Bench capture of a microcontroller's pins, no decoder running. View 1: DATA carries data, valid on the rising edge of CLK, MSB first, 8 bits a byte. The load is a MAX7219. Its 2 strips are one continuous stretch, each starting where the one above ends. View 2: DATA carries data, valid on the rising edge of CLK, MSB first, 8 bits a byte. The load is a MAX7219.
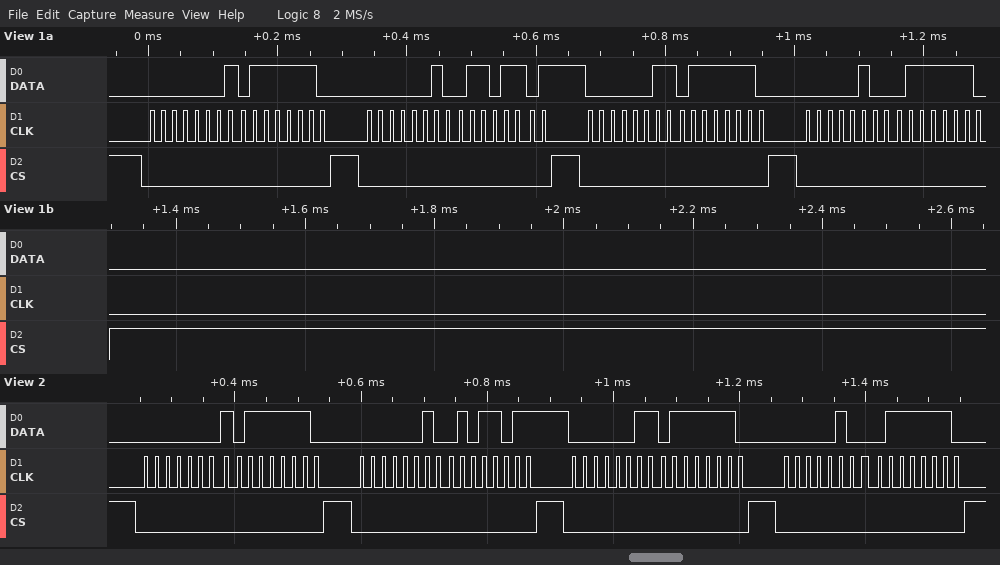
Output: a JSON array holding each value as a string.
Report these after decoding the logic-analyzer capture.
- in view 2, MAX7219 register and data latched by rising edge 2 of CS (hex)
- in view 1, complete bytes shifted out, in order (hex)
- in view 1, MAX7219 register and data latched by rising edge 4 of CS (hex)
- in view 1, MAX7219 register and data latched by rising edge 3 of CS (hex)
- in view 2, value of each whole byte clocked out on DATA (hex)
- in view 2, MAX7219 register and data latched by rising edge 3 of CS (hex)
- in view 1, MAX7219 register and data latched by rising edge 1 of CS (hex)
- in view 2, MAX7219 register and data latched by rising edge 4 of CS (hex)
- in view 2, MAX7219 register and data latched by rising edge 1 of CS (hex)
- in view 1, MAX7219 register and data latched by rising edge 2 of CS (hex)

["register 0x2, data 0x5B", "01 7E 02 6D 03 7E 04 7E", "register 0x4, data 0x7E", "register 0x3, data 0x7E", "01 7E 02 5B 03 7E 04 7E", "register 0x3, data 0x7E", "register 0x1, data 0x7E", "register 0x4, data 0x7E", "register 0x1, data 0x7E", "register 0x2, data 0x6D"]
